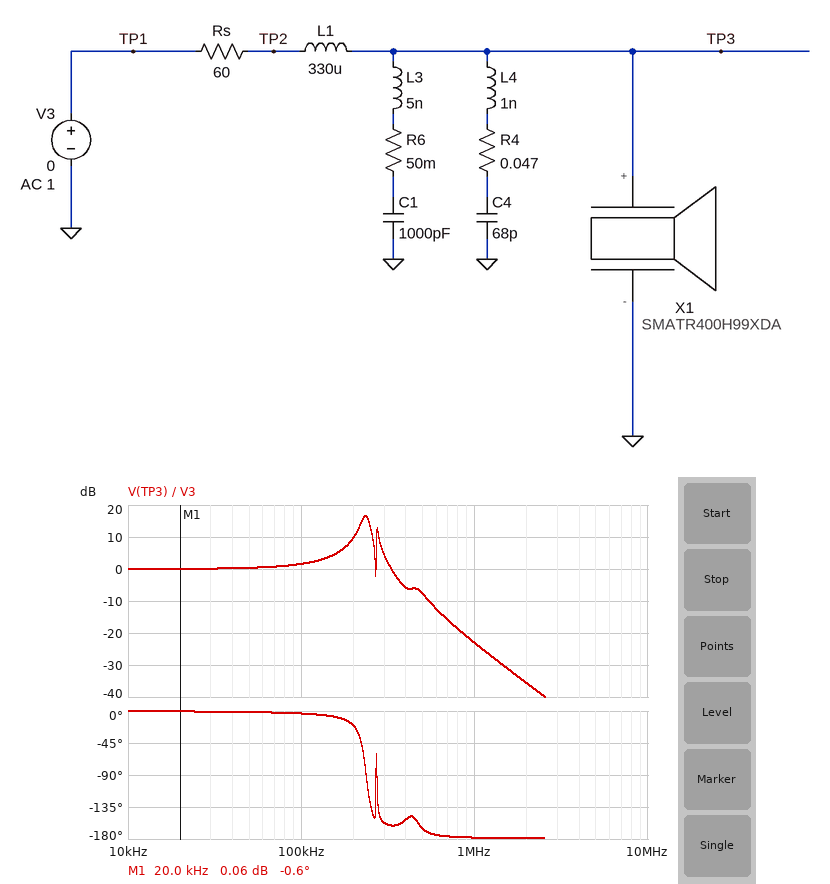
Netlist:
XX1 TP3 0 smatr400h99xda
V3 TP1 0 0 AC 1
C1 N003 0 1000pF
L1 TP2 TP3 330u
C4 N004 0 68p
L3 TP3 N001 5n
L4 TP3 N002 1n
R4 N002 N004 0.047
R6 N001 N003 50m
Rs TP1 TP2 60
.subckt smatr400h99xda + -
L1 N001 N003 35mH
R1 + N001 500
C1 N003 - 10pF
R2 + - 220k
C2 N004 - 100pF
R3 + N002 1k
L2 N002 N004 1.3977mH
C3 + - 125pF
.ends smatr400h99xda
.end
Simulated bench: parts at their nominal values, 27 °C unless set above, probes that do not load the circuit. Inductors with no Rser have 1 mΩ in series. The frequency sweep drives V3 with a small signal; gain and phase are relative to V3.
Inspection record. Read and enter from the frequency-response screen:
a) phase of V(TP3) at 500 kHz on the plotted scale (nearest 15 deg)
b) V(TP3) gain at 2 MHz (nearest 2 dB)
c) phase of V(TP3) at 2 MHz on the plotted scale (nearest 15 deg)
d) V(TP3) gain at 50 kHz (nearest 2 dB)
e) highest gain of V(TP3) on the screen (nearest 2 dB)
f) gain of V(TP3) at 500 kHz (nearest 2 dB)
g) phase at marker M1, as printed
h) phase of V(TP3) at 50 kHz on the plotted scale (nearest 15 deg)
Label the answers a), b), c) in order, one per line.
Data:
a) -165 deg
b) -36 dB
c) -180 deg
d) 0 dB
e) 16 dB
f) -8 dB
g) -0.6 deg
h) 0 deg
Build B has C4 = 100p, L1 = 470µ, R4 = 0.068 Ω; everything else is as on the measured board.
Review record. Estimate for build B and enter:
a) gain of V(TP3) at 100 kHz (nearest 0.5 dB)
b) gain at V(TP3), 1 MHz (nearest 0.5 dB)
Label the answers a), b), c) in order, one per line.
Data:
a) 2.5 dB
b) -26.5 dB
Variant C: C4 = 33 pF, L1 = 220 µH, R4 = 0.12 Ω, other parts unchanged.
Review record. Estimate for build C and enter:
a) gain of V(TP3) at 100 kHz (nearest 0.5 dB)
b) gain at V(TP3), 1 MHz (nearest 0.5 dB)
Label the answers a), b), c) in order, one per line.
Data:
a) 1.0 dB
b) -19.0 dB
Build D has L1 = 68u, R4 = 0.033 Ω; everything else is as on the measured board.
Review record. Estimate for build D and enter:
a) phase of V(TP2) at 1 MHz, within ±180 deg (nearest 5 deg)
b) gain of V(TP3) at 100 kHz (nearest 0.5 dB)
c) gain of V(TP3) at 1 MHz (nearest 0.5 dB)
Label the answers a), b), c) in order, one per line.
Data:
a) 10 deg
b) 0.5 dB
c) -7.0 dB
